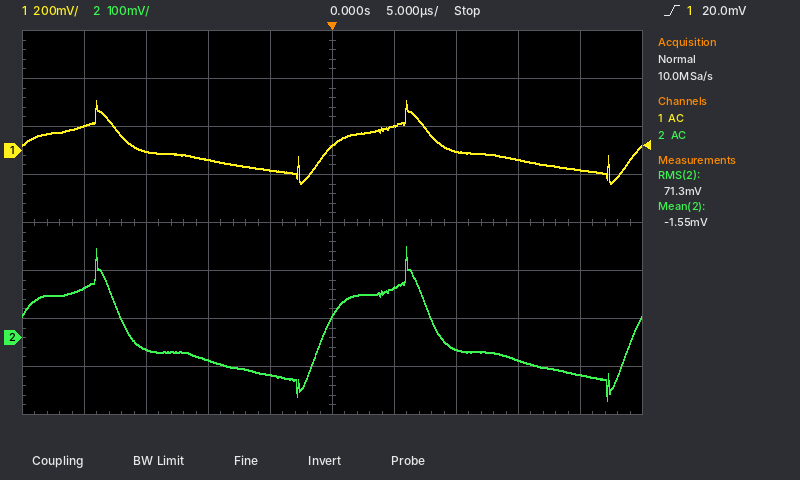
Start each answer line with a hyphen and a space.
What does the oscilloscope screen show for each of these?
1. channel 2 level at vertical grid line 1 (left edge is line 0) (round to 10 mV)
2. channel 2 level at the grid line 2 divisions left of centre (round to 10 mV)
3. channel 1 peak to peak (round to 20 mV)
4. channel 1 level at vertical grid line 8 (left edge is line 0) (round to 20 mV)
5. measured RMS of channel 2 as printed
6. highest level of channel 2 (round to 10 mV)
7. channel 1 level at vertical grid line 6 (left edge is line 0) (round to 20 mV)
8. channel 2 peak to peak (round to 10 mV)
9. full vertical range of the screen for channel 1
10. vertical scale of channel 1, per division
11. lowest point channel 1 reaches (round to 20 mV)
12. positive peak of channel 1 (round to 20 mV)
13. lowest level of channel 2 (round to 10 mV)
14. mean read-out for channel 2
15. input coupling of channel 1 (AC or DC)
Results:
- 100 mV
- -50 mV
- 340 mV
- -40 mV
- 71.3 mV
- 190 mV
- 100 mV
- 320 mV
- 1.6 V
- 200 mV
- -140 mV
- 200 mV
- -130 mV
- -1.55 mV
- AC
